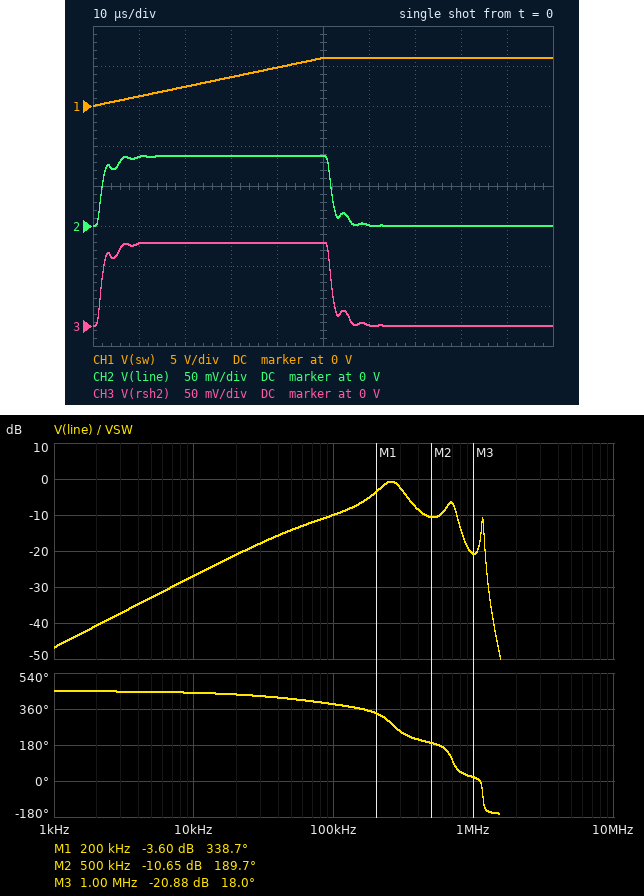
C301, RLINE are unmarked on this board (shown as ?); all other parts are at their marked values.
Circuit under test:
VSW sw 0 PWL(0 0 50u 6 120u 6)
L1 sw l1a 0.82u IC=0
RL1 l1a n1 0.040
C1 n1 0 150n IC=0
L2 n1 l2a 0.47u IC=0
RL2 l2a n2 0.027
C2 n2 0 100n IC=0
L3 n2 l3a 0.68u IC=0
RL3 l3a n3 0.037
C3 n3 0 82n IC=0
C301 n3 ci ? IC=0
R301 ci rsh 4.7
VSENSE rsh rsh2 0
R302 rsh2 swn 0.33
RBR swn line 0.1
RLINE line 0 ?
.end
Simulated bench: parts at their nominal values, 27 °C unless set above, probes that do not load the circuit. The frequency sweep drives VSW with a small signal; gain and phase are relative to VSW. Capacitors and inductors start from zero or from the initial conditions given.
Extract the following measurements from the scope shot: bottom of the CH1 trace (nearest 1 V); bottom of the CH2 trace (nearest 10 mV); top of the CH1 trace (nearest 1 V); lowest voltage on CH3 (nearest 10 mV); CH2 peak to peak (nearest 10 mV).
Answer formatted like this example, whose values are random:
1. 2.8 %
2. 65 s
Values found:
1. 0 V
2. 0 V
3. 6 V
4. 0 V
5. 90 mV
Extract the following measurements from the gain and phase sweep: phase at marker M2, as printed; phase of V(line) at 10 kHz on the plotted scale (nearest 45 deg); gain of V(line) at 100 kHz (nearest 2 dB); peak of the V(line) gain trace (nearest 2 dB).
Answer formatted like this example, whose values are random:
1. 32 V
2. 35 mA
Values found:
1. 189.7 deg
2. 450 deg
3. -10 dB
4. 0 dB
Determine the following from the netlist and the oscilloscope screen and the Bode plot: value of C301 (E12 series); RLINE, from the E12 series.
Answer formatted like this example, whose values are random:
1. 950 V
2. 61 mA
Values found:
1. 330 nF
2. 2.2 Ω
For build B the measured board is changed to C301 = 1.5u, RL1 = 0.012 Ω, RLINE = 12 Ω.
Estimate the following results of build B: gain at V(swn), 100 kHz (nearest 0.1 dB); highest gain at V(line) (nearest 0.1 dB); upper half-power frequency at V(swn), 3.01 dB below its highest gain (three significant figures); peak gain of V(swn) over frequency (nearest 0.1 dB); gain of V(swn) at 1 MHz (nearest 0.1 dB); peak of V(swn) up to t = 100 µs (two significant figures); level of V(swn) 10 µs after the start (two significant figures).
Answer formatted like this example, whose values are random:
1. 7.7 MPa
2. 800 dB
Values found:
1. -1.6 dB
2. 13.7 dB
3. 295 kHz
4. 13.8 dB
5. -13.0 dB
6. 1.9 V
7. 710 mV
